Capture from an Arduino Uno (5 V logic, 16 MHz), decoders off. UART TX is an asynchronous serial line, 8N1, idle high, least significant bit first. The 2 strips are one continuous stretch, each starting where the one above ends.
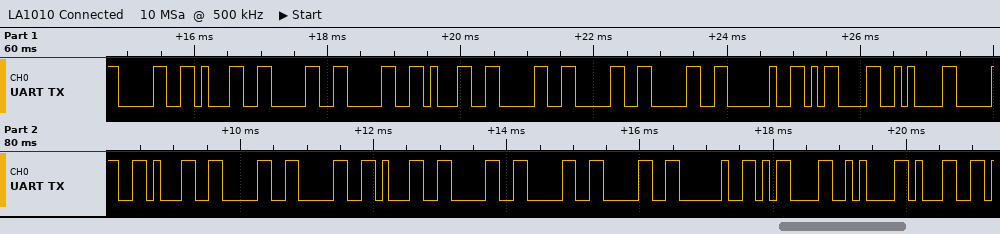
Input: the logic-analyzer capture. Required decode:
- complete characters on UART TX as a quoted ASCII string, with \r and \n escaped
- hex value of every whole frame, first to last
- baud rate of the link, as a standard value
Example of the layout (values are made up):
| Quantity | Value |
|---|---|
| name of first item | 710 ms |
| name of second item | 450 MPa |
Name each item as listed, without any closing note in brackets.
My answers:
| Quantity | Value |
|---|---|
| complete characters on UART TX as a quoted ASCII string, with \r and \n escaped | "01001000 \r\n01001000 \r\n1" |
| hex value of every whole frame, first to last | 30 31 30 30 31 30 30 30 20 0D 0A 30 31 30 30 31 30 30 30 20 0D 0A 31 |
| baud rate of the link, as a standard value | 9600 baud |
